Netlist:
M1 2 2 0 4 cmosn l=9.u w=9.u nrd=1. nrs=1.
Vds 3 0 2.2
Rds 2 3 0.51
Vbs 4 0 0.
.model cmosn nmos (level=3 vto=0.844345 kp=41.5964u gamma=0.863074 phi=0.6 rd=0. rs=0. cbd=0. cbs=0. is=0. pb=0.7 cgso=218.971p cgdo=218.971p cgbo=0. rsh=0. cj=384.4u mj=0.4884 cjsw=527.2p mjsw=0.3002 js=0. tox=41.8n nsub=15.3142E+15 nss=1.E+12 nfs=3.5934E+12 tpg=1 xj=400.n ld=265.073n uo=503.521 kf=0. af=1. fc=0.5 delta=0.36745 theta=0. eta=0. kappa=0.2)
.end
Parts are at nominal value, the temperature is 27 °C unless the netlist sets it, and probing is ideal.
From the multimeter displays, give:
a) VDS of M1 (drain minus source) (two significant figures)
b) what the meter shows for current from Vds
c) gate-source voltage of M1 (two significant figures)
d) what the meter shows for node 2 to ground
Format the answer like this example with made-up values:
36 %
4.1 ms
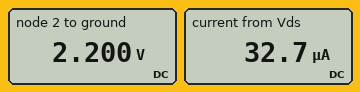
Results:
2.2 V
32.7 µA
2.2 V
2.200 V
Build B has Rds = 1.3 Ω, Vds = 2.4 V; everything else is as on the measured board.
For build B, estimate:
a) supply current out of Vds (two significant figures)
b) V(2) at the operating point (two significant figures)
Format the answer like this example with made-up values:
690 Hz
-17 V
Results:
43 µA
2.4 V
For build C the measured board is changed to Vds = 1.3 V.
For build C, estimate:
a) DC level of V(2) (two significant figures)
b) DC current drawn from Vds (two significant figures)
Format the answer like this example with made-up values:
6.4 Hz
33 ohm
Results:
1.3 V
3.8 µA
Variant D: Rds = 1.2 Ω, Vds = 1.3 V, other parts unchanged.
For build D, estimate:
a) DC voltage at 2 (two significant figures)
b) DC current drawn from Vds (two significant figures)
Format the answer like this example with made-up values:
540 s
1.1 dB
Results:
1.3 V
3.8 µA
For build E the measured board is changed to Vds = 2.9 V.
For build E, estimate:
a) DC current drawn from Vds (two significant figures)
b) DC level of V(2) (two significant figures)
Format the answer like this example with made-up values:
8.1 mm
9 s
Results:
75 µA
2.9 V
